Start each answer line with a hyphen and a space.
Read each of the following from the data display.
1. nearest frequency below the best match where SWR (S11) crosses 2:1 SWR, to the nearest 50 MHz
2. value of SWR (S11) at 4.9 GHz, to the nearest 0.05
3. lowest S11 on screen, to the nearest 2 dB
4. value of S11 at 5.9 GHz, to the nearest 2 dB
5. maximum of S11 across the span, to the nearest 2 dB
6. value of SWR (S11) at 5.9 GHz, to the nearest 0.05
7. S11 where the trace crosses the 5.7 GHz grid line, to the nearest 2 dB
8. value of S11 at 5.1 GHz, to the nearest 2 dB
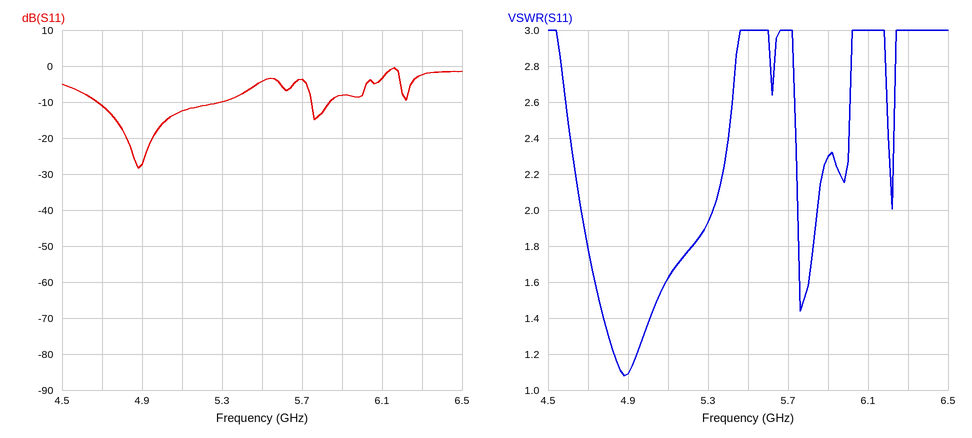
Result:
- 4.65 GHz
- 1.10
- -28 dB
- -8 dB
- 0 dB
- 2.30
- -4 dB
- -12 dB
